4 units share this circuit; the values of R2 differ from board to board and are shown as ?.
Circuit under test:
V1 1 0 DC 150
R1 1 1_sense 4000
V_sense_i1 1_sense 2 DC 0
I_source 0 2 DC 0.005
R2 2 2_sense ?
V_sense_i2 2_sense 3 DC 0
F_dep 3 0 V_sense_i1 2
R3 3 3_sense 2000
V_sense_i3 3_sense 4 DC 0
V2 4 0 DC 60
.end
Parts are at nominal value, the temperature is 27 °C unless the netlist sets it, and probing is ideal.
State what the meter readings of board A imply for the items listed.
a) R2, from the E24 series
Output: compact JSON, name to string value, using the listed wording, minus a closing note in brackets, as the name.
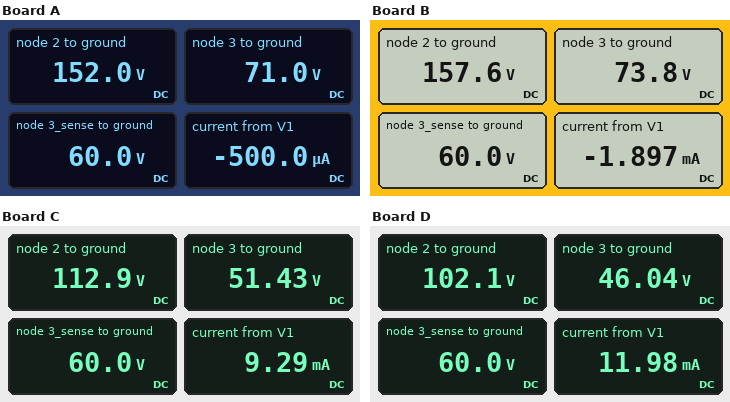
{"R2, from the E24 series": "18 kΩ"}
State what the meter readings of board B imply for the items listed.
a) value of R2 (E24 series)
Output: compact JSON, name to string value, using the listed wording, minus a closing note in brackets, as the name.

{"value of R2": "27 kΩ"}
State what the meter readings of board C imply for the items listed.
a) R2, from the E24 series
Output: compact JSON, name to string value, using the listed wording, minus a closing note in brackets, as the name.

{"R2, from the E24 series": "4.3 kΩ"}
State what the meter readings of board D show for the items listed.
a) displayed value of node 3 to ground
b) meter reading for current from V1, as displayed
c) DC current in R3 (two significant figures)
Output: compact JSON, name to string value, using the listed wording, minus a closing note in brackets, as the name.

{"displayed value of node 3 to ground": "46.04 V", "meter reading for current from V1, as displayed": "11.98 mA", "DC current in R3": "7.0 mA"}
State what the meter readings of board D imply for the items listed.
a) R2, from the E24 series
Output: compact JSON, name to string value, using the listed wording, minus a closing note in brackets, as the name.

{"R2, from the E24 series": "3.3 kΩ"}
